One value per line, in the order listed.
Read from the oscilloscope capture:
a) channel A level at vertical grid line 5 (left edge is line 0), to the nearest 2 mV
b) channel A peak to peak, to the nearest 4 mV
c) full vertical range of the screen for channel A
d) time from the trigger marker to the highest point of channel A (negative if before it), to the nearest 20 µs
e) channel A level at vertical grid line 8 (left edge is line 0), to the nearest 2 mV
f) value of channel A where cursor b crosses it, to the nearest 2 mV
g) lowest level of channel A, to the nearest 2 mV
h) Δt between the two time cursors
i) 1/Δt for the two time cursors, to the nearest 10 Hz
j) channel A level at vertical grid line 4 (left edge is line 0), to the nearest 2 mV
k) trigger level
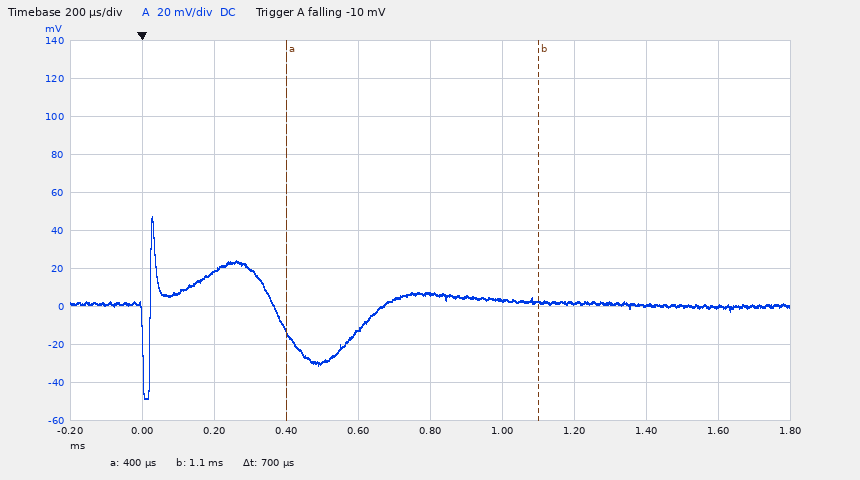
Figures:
6 mV
96 mV
200 mV
+20 µs
0 mV
2 mV
-48 mV
700 µs
1.43 kHz
-12 mV
-10 mV
